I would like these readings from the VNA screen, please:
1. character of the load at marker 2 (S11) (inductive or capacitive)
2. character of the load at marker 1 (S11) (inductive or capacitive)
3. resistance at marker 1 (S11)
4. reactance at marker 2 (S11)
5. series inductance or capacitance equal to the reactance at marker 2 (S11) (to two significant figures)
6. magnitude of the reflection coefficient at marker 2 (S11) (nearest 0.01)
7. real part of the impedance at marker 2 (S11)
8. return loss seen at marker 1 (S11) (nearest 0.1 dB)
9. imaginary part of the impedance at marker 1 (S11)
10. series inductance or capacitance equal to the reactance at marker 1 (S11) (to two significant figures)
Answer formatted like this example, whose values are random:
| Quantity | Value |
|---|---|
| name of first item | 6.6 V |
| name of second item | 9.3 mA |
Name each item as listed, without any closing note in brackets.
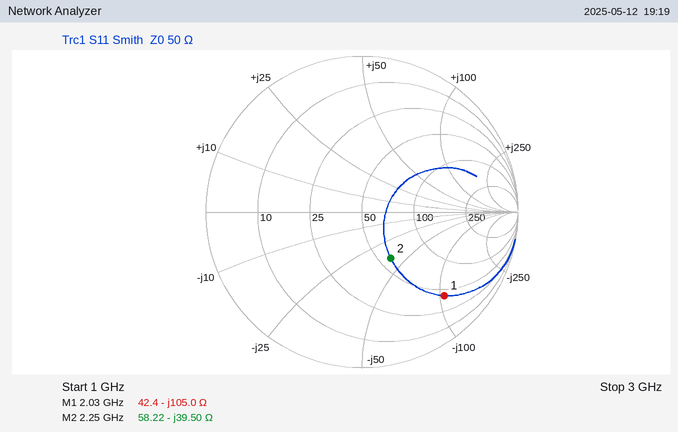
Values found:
| Quantity | Value |
|---|---|
| character of the load at marker 2 (S11) | capacitive |
| character of the load at marker 1 (S11) | capacitive |
| resistance at marker 1 | 42.4 Ω |
| reactance at marker 2 | -39.50 Ω |
| series inductance or capacitance equal to the reactance at marker 2 (S11) | 1.8 pF |
| magnitude of the reflection coefficient at marker 2 (S11) | 0.35 |
| real part of the impedance at marker 2 | 58.22 Ω |
| return loss seen at marker 1 (S11) | 2.5 dB |
| imaginary part of the impedance at marker 1 | -105.0 Ω |
| series inductance or capacitance equal to the reactance at marker 1 (S11) | 750 fF |
